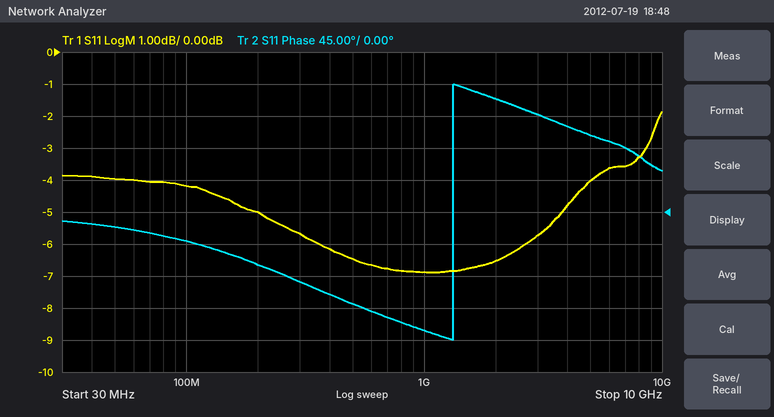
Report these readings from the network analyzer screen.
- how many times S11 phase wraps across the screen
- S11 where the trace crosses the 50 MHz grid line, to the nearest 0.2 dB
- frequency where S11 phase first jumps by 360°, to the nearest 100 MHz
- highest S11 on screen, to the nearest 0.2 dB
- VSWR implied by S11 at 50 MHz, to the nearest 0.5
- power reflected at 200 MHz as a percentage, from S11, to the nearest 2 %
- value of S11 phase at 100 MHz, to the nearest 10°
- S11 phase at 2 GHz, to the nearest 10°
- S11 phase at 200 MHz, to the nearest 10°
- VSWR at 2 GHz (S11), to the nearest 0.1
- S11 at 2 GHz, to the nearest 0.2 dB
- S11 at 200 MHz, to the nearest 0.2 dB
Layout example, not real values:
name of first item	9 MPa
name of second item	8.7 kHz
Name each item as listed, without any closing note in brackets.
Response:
how many times S11 phase wraps across the screen	1
S11 where the trace crosses the 50 MHz grid line, to the nearest 0.2 dB	-4.0 dB
frequency where S11 phase first jumps by 360°, to the nearest 100 MHz	1.3 GHz
highest S11 on screen, to the nearest 0.2 dB	-1.8 dB
VSWR implied by S11 at 50 MHz, to the nearest 0.5	4.5
power reflected at 200 MHz as a percentage, from S11, to the nearest 2 %	32 %
value of S11 phase at 100 MHz, to the nearest 10°	-40°
S11 phase at 2 GHz, to the nearest 10°	160°
S11 phase at 200 MHz, to the nearest 10°	-70°
VSWR at 2 GHz (S11), to the nearest 0.1	2.8
S11 at 2 GHz, to the nearest 0.2 dB	-6.6 dB
S11 at 200 MHz, to the nearest 0.2 dB	-5.0 dB
